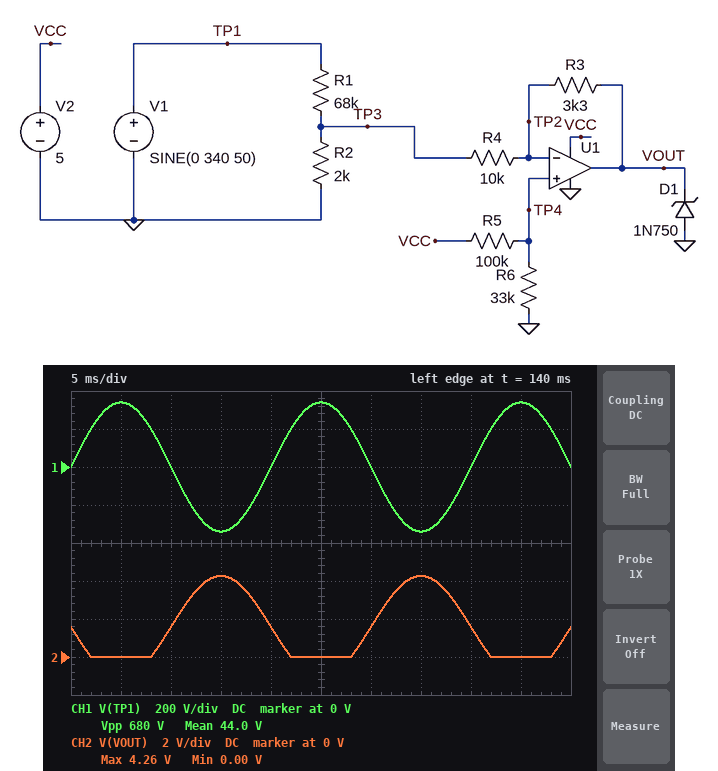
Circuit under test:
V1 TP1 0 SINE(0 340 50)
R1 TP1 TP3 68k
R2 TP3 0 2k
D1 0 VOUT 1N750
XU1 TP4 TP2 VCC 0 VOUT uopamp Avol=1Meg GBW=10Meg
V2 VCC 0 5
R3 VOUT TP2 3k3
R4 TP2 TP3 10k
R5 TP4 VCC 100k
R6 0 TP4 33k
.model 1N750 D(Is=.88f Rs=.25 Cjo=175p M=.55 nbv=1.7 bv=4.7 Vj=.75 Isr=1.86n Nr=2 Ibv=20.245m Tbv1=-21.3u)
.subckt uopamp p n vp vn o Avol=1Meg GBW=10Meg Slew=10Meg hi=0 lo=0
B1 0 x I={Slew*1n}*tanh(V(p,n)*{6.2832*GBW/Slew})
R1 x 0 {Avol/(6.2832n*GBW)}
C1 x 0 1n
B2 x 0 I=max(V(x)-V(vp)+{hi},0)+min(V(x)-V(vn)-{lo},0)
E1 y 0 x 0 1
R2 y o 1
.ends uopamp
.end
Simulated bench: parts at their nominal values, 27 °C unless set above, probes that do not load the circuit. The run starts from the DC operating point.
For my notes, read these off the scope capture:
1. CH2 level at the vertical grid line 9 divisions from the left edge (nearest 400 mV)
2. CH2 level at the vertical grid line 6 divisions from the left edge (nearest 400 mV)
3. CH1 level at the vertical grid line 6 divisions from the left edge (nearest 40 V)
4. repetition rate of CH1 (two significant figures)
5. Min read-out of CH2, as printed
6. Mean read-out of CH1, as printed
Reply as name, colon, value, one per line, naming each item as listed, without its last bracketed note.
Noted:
CH2 level at the vertical grid line 9 divisions from the left edge: 0 V
CH2 level at the vertical grid line 6 divisions from the left edge: 1.6 V
CH1 level at the vertical grid line 6 divisions from the left edge: 0 V
repetition rate of CH1: 50 Hz
Min read-out of CH2, as printed: 0.00 V
Mean read-out of CH1, as printed: 44.0 V
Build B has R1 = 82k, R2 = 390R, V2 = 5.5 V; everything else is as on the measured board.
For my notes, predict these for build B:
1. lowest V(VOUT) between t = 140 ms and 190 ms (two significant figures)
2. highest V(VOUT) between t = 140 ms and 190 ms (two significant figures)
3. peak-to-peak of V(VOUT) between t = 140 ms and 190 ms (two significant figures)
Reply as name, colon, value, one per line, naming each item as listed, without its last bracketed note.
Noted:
lowest V(VOUT) between t = 140 ms and 190 ms: 1.3 V
highest V(VOUT) between t = 140 ms and 190 ms: 2.3 V
peak-to-peak of V(VOUT) between t = 140 ms and 190 ms: 1.0 V
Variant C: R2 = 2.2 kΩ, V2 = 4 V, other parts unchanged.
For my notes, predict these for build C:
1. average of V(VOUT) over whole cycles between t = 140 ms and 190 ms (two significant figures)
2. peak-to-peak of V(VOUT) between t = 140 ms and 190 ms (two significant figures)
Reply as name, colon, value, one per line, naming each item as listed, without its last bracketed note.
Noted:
average of V(VOUT) over whole cycles between t = 140 ms and 190 ms: 1.6 V
peak-to-peak of V(VOUT) between t = 140 ms and 190 ms: 4.0 V
